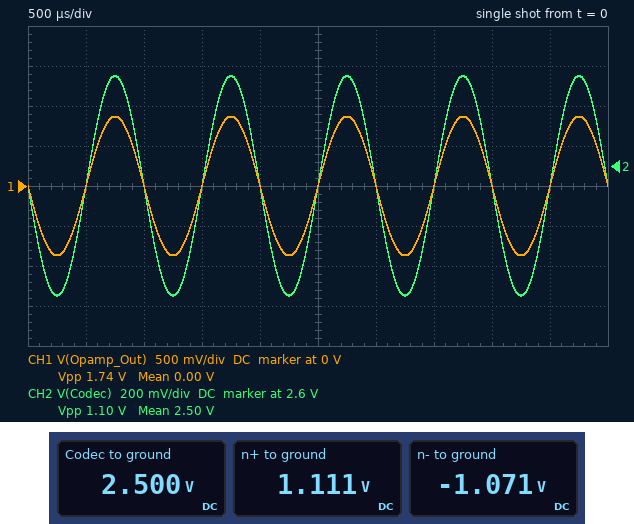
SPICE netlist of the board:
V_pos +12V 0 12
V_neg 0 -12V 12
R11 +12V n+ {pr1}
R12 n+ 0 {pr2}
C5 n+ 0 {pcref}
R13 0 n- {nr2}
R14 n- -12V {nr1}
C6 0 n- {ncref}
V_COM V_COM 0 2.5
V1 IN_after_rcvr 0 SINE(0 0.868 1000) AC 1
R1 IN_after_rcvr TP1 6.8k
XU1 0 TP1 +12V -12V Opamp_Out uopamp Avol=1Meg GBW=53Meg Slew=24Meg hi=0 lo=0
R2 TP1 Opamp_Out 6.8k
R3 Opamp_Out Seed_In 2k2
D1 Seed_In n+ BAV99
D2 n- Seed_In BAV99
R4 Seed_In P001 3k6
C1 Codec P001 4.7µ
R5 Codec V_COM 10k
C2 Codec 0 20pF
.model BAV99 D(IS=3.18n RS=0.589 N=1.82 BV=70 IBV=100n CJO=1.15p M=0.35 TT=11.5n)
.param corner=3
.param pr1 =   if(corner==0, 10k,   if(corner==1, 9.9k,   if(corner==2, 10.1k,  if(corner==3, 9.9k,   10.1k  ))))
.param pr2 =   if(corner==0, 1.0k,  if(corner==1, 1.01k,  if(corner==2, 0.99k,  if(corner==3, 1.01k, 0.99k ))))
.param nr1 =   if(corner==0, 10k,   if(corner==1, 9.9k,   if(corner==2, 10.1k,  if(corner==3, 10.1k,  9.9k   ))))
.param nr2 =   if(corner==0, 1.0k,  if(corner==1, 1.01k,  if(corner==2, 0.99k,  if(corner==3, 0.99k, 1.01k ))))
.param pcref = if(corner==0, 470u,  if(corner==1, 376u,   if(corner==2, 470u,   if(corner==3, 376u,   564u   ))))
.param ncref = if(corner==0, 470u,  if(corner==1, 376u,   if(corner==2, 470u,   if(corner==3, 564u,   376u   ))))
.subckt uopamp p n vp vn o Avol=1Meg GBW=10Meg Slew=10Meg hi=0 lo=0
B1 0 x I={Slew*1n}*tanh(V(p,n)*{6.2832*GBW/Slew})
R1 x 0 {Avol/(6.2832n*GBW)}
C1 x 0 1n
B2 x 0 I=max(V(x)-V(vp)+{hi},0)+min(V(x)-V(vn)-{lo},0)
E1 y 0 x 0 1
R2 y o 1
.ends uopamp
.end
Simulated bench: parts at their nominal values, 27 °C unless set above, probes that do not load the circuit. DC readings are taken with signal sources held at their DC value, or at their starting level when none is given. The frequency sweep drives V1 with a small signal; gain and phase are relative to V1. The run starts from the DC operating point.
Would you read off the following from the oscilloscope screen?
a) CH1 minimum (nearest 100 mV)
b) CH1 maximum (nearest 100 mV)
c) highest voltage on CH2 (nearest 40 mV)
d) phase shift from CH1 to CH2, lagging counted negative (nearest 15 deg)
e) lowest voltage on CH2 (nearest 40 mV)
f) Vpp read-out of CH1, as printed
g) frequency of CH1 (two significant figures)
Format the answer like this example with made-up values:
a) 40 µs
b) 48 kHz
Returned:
a) -900 mV
b) 900 mV
c) 3.04 V
d) 0 deg
e) 1.96 V
f) 1.74 V
g) 1.0 kHz
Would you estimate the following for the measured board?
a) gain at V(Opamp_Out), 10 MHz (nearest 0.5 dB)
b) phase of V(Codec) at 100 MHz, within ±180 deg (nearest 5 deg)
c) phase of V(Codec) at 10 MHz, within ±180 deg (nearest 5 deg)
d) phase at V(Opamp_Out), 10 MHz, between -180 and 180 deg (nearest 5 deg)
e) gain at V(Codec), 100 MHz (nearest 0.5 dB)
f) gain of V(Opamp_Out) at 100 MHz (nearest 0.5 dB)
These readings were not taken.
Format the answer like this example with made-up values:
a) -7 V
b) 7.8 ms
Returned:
a) -0.5 dB
b) -40 deg
c) 75 deg
d) 160 deg
e) -54.5 dB
f) -12.0 dB
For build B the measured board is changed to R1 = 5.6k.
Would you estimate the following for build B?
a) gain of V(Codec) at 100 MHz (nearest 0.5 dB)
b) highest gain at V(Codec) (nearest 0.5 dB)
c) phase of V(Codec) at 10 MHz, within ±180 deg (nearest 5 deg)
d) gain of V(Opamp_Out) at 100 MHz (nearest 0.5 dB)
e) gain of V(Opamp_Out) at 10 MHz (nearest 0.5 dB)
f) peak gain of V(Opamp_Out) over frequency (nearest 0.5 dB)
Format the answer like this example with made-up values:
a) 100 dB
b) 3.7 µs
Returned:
a) -53.5 dB
b) -2.5 dB
c) 70 deg
d) -11.0 dB
e) 1.0 dB
f) 1.5 dB
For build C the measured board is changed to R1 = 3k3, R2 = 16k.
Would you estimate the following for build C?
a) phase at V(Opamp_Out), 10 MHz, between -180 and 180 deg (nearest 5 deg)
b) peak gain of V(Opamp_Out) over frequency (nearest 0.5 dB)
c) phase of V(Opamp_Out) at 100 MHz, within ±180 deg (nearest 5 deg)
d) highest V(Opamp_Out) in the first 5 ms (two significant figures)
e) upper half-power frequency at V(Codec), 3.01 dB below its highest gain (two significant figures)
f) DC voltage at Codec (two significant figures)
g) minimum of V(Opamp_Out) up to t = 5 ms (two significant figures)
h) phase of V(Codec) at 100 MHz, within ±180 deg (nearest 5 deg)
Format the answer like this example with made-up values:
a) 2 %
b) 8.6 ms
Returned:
a) 130 deg
b) 13.5 dB
c) 95 deg
d) 4.2 V
e) 2.0 MHz
f) 2.5 V
g) -4.2 V
h) -50 deg
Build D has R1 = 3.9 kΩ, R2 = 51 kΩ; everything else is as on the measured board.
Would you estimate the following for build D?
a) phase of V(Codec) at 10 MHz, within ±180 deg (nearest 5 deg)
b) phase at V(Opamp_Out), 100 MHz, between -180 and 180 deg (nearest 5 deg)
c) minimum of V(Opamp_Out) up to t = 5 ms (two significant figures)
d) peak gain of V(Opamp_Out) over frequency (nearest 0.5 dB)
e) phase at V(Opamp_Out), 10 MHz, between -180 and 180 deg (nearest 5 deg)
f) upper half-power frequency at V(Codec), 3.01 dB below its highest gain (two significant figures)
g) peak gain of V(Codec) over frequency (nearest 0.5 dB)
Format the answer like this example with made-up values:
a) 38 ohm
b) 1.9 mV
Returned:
a) 25 deg
b) 90 deg
c) -11 V
d) 22.5 dB
e) 110 deg
f) 1.7 MHz
g) 18.5 dB
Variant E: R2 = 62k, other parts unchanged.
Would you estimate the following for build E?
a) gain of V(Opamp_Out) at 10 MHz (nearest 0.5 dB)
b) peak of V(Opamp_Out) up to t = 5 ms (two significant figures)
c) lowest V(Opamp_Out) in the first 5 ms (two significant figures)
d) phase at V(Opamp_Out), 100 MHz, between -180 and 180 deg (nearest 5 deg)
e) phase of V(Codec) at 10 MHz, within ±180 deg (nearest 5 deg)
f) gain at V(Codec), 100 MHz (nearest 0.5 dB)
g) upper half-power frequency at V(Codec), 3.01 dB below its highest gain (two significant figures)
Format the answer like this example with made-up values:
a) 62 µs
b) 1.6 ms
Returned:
a) 12.5 dB
b) 7.9 V
c) -7.9 V
d) 95 deg
e) 30 deg
f) -49.0 dB
g) 1.9 MHz
